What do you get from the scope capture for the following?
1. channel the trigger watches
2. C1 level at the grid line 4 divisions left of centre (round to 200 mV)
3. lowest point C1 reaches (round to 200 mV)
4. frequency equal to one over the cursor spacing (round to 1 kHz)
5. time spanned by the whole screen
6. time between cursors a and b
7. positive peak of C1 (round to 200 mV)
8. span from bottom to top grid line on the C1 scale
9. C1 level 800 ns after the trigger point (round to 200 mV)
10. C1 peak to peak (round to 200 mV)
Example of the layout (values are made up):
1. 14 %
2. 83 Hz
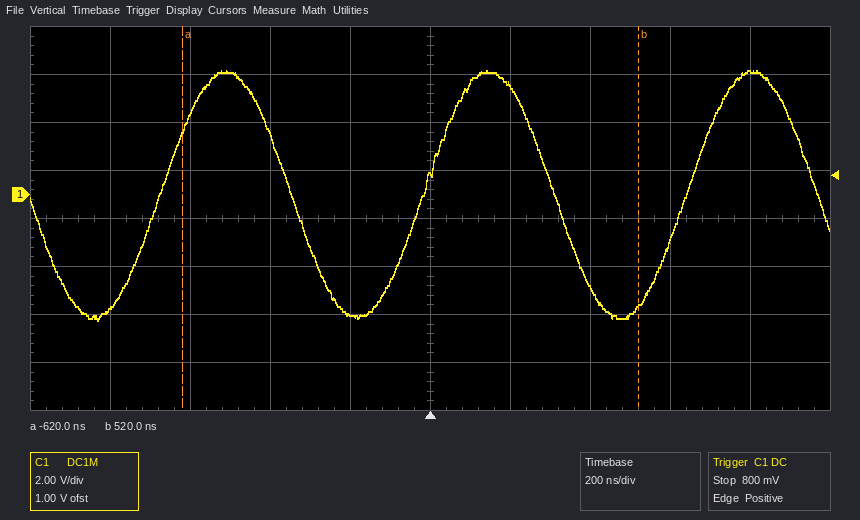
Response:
1. C1
2. -4.8 V
3. -5.2 V
4. 877 kHz
5. 2 µs
6. 1.14 µs
7. 5.2 V
8. 16 V
9. 5.2 V
10. 10.4 V
